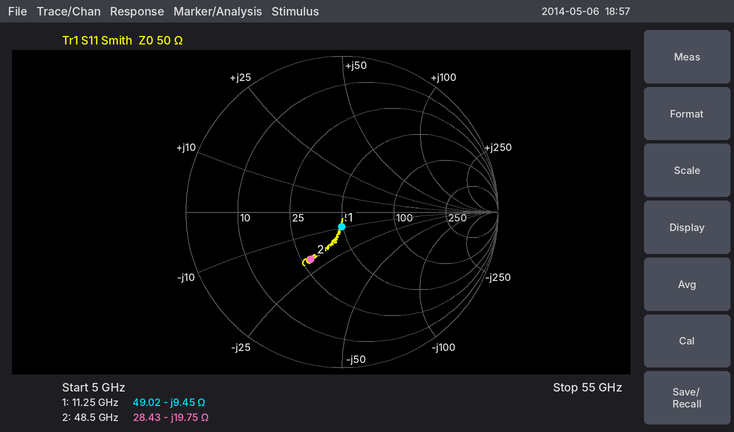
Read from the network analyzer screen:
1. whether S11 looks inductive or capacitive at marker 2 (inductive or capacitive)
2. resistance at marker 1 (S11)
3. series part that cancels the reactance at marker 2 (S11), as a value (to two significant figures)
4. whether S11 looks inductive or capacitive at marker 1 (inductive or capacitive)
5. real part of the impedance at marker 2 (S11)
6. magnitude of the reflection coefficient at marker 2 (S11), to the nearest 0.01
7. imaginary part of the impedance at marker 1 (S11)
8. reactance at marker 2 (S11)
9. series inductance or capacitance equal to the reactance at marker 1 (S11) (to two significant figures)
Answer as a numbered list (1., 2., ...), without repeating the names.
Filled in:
1. capacitive
2. 49.02 Ω
3. 65 pH
4. capacitive
5. 28.43 Ω
6. 0.36
7. -9.45 Ω
8. -19.75 Ω
9. 1.5 pF
